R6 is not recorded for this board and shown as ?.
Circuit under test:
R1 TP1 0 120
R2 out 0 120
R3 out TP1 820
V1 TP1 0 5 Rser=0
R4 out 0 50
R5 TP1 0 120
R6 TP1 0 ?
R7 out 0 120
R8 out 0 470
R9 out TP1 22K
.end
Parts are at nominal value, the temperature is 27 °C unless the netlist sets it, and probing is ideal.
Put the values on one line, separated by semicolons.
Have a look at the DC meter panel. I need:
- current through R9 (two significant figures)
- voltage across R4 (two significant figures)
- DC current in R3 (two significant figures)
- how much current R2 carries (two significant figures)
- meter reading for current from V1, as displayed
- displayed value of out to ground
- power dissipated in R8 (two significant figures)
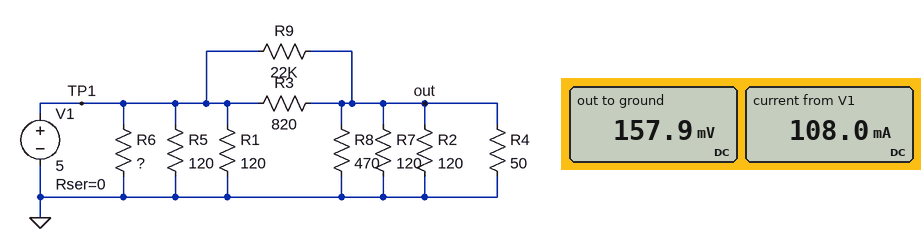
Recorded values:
220 µA; 160 mV; 5.9 mA; 1.3 mA; 108.0 mA; 157.9 mV; 53 µW
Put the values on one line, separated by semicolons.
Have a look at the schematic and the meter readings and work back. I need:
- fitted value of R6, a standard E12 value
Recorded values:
270 Ω
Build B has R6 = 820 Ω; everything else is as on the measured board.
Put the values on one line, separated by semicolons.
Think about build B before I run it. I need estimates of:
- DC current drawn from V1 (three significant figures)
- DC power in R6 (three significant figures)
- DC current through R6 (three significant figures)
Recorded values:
95.6 mA; 30.5 mW; 6.10 mA
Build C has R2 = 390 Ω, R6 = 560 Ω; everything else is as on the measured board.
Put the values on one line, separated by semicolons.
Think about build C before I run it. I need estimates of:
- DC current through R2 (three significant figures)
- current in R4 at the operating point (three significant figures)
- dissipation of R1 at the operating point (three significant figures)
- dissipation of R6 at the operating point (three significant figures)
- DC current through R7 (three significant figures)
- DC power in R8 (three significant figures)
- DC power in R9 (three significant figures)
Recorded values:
473 µA; 3.69 mA; 208 mW; 44.6 mW; 1.54 mA; 72.4 µW; 1.05 mW
